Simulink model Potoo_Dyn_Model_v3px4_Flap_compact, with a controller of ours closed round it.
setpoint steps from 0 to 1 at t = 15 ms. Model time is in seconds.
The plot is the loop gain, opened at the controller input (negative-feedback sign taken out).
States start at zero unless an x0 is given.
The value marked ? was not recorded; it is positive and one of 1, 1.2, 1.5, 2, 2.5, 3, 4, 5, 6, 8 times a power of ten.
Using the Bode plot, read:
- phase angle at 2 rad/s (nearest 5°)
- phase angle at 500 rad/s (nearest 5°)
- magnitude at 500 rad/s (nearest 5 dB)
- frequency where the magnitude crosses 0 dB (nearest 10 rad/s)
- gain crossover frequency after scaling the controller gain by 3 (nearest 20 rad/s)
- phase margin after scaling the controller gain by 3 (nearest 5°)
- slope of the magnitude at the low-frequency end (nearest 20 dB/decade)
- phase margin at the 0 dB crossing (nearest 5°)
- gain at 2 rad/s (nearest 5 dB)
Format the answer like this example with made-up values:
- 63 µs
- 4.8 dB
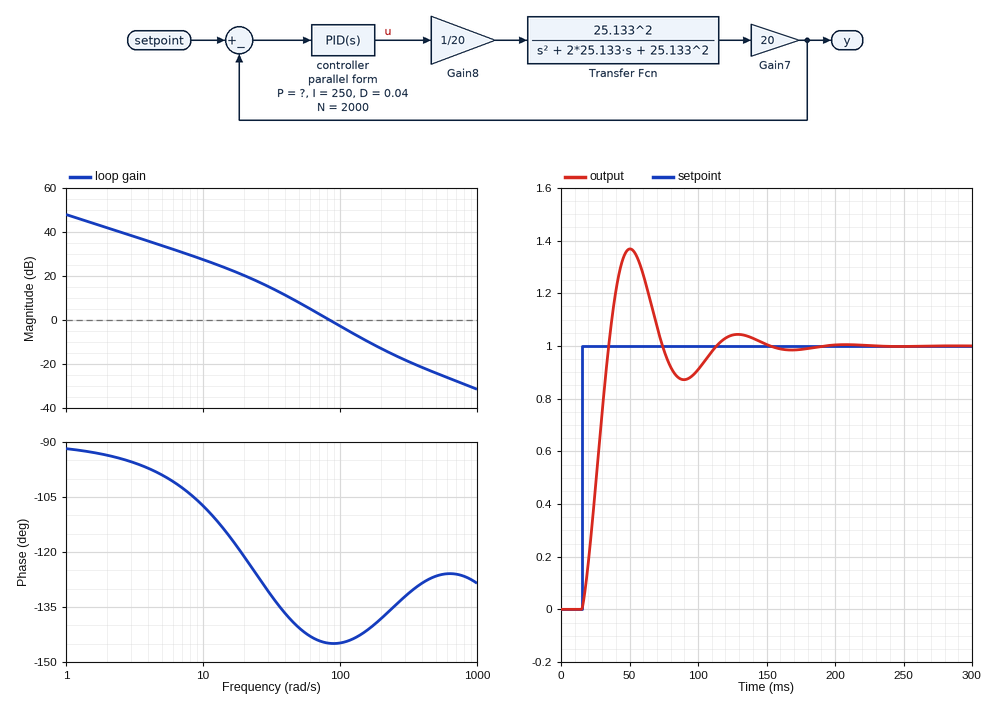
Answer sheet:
- -95°
- -125°
- -25 dB
- 80 rad/s
- 160 rad/s
- 40°
- -20 dB/decade
- 35°
- 40 dB
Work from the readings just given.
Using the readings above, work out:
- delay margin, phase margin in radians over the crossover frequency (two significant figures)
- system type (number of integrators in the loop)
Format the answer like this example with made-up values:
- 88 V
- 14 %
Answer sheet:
- 0.0076 s
- 1
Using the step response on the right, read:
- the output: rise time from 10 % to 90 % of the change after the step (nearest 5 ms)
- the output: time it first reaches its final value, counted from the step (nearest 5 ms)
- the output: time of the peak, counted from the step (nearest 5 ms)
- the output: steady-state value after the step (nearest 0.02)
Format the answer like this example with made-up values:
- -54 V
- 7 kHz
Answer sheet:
- 15 ms
- 20 ms
- 35 ms
- 1.00
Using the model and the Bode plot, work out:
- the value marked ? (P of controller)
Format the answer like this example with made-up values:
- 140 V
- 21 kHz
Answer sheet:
- 12
